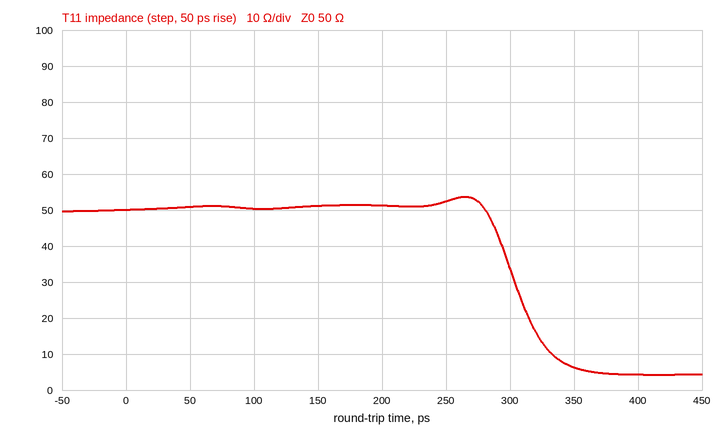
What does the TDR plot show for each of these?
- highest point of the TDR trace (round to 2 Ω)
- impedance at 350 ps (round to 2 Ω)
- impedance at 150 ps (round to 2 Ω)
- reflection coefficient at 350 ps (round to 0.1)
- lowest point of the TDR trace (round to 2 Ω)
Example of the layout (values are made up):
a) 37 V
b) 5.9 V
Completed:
a) 54 Ω
b) 6 Ω
c) 52 Ω
d) -0.8
e) 4 Ω
